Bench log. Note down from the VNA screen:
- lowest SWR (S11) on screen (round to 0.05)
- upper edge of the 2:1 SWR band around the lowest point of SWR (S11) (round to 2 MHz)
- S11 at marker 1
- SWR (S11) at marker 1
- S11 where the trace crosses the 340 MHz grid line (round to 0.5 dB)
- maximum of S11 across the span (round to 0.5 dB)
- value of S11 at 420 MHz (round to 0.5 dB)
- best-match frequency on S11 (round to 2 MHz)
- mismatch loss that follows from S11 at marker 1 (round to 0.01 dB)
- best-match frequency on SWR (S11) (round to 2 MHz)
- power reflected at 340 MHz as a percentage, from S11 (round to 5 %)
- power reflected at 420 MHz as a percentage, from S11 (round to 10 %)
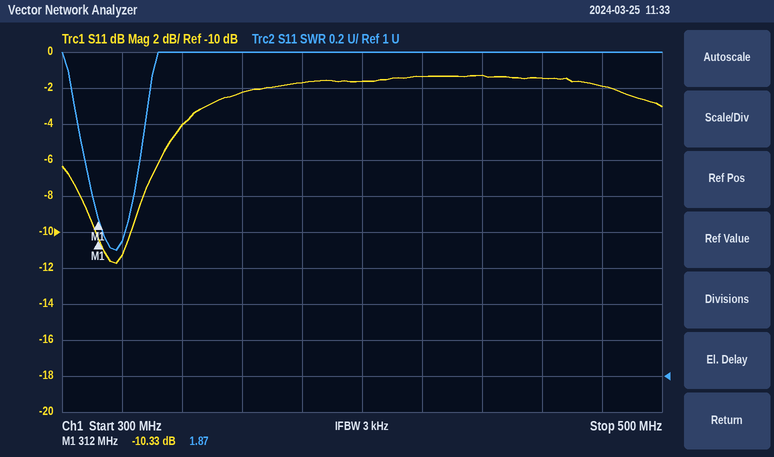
1.70
324 MHz
-10.33 dB
1.87
-4.0 dB
-1.5 dB
-1.5 dB
318 MHz
0.42 dB
318 MHz
40 %
70 %
